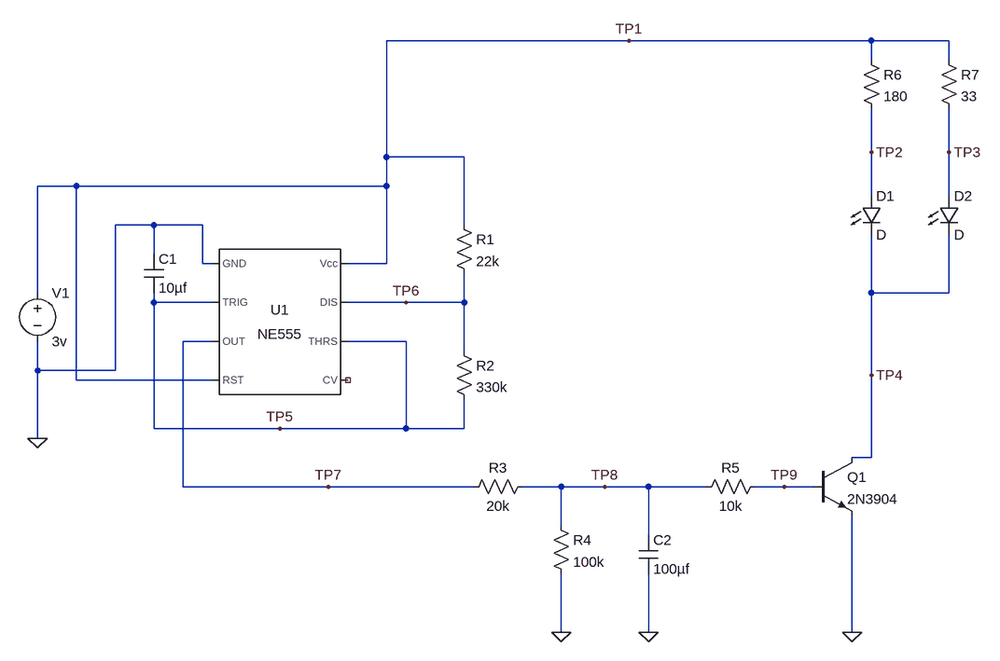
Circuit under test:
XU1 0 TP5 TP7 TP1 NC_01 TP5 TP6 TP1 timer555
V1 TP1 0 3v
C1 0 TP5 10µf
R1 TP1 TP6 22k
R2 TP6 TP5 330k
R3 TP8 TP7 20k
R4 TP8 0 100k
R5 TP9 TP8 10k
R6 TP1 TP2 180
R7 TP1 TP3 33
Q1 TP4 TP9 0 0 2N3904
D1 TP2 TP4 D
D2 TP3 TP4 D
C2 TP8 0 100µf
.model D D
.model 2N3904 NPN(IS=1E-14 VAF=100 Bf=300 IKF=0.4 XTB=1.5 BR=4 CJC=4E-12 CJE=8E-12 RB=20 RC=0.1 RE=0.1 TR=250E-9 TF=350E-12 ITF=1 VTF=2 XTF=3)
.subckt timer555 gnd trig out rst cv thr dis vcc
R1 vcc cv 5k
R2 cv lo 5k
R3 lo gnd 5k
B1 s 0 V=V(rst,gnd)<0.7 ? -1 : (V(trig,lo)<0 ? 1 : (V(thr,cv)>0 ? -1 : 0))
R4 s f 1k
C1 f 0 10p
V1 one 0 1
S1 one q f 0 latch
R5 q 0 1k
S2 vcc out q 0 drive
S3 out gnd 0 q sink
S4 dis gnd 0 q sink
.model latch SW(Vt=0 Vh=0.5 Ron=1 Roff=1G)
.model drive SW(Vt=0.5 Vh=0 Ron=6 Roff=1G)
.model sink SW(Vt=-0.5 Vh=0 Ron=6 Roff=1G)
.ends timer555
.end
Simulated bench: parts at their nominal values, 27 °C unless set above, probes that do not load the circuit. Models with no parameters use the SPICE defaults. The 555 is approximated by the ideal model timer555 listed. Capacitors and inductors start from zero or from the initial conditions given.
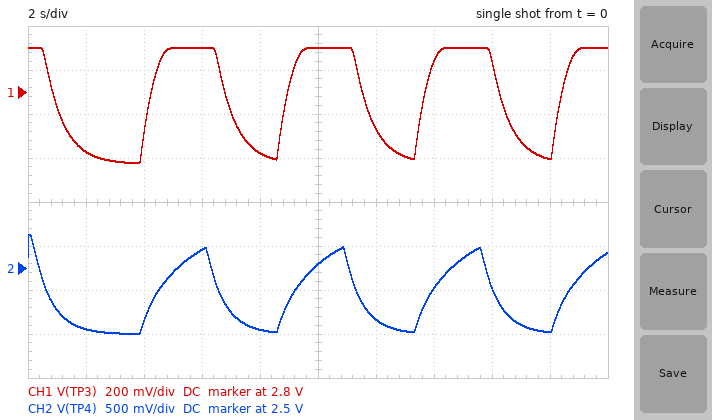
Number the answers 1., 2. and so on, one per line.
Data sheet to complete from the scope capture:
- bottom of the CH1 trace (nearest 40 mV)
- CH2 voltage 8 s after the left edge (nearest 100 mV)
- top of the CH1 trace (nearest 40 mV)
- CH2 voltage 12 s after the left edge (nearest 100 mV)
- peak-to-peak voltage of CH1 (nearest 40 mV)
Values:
1. 2.48 V
2. 1.8 V
3. 3.00 V
4. 1.9 V
5. 520 mV
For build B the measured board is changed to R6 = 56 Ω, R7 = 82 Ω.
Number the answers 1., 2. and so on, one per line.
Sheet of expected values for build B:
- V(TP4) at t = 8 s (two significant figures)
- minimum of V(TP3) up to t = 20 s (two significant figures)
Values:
1. 1.7 V
2. 2.4 V
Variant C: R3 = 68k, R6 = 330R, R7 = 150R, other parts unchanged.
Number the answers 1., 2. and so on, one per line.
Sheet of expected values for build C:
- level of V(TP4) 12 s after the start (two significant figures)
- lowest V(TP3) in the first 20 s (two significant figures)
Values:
1. 2.1 V
2. 2.4 V
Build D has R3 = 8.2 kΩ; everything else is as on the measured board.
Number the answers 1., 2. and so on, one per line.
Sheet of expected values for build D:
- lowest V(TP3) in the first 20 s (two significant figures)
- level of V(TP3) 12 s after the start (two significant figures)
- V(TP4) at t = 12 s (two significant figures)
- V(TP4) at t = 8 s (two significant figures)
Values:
1. 2.1 V
2. 2.2 V
3. 1.5 V
4. 1.4 V
